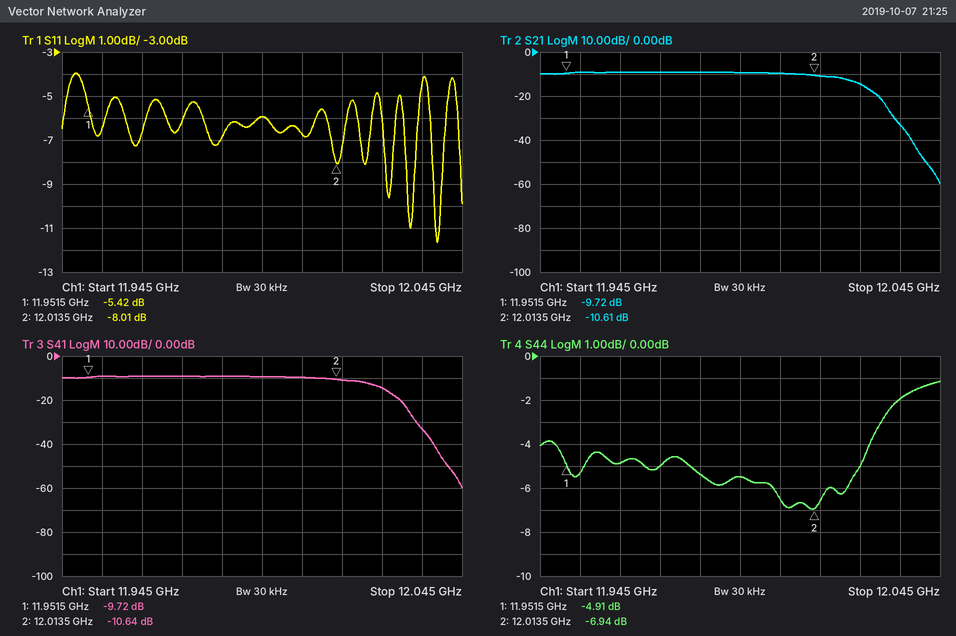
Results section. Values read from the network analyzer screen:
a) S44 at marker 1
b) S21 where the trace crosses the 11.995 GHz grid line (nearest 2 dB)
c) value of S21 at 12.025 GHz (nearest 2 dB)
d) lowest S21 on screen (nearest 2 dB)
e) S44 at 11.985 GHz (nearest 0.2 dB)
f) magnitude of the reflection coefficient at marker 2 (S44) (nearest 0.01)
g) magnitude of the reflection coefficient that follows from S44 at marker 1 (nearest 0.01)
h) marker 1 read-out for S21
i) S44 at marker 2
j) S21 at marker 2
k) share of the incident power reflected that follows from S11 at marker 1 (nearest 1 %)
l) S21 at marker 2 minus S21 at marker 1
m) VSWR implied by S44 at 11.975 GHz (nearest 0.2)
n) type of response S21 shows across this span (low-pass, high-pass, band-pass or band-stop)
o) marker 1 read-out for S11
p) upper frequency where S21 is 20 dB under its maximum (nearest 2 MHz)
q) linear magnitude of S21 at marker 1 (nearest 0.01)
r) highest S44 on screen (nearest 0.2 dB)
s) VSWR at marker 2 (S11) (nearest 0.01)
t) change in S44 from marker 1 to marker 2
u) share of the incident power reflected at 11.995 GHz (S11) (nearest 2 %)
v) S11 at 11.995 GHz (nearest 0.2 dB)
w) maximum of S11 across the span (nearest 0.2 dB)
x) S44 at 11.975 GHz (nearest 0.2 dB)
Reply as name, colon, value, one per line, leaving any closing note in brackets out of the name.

S44 at marker 1: -4.91 dB
S21 where the trace crosses the 11.995 GHz grid line: -10 dB
value of S21 at 12.025 GHz: -14 dB
lowest S21 on screen: -60 dB
S44 at 11.985 GHz: -5.4 dB
magnitude of the reflection coefficient at marker 2 (S44): 0.45
magnitude of the reflection coefficient that follows from S44 at marker 1: 0.57
marker 1 read-out for S21: -9.72 dB
S44 at marker 2: -6.94 dB
S21 at marker 2: -10.61 dB
share of the incident power reflected that follows from S11 at marker 1: 29 %
S21 at marker 2 minus S21 at marker 1: -0.89 dB
VSWR implied by S44 at 11.975 GHz: 3.6
type of response S21 shows across this span: low-pass
marker 1 read-out for S11: -5.42 dB
upper frequency where S21 is 20 dB under its maximum: 12.034 GHz
linear magnitude of S21 at marker 1: 0.33
highest S44 on screen: -1.2 dB
VSWR at marker 2 (S11): 2.32
change in S44 from marker 1 to marker 2: -2.03 dB
share of the incident power reflected at 11.995 GHz (S11): 26 %
S11 at 11.995 GHz: -6.0 dB
maximum of S11 across the span: -4.0 dB
S44 at 11.975 GHz: -5.0 dB
